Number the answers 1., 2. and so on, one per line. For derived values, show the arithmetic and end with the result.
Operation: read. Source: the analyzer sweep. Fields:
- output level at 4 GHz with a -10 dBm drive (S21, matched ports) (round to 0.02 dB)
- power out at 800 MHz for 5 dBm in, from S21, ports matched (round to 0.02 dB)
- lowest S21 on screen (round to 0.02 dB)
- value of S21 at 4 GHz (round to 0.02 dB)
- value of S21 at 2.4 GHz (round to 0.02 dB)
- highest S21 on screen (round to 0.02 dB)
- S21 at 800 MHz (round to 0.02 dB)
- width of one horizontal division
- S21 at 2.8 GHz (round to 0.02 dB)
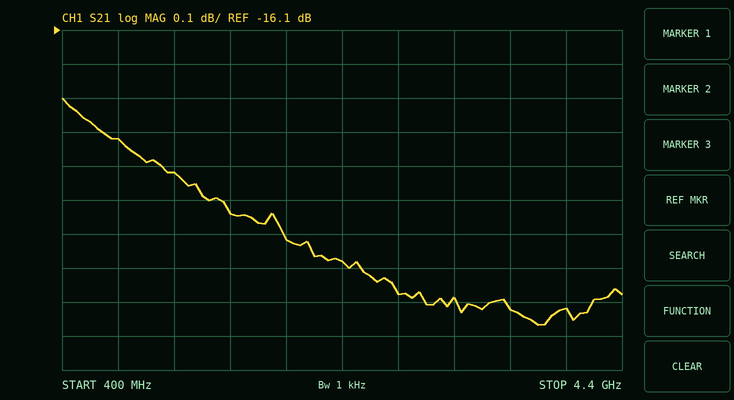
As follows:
1. -10 dBm + (-16.92 dB) = -26.92 dBm
2. 5 dBm + (-16.42 dB) = -11.42 dBm
3. -16.96 dB
4. -16.92 dB
5. -16.78 dB
6. -16.30 dB
7. -16.42 dB
8. 400 MHz
9. -16.88 dB
